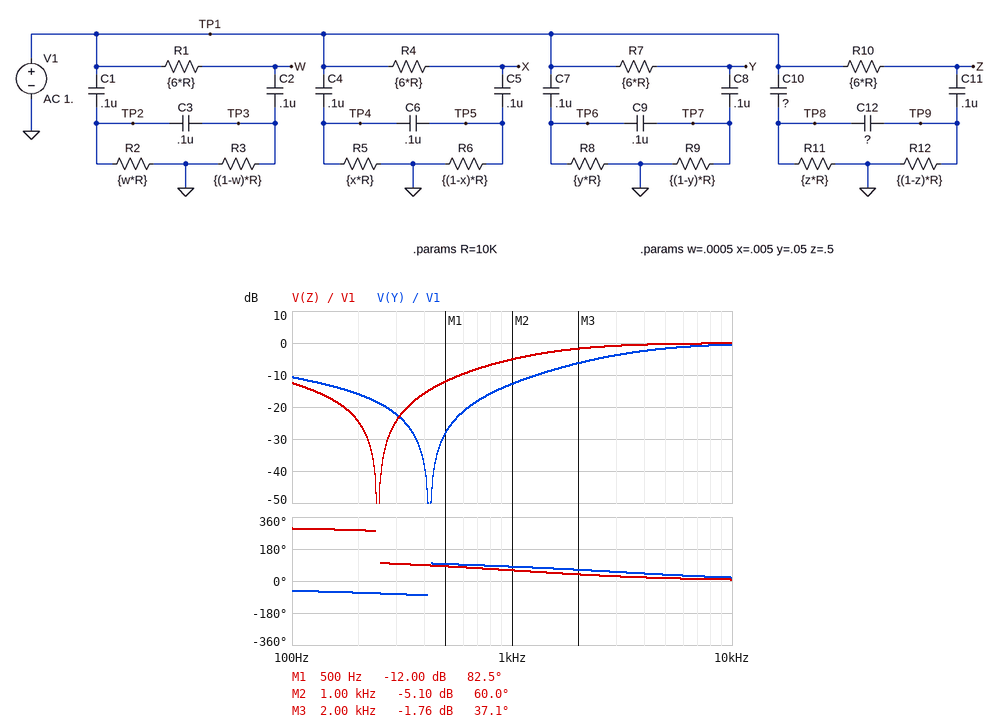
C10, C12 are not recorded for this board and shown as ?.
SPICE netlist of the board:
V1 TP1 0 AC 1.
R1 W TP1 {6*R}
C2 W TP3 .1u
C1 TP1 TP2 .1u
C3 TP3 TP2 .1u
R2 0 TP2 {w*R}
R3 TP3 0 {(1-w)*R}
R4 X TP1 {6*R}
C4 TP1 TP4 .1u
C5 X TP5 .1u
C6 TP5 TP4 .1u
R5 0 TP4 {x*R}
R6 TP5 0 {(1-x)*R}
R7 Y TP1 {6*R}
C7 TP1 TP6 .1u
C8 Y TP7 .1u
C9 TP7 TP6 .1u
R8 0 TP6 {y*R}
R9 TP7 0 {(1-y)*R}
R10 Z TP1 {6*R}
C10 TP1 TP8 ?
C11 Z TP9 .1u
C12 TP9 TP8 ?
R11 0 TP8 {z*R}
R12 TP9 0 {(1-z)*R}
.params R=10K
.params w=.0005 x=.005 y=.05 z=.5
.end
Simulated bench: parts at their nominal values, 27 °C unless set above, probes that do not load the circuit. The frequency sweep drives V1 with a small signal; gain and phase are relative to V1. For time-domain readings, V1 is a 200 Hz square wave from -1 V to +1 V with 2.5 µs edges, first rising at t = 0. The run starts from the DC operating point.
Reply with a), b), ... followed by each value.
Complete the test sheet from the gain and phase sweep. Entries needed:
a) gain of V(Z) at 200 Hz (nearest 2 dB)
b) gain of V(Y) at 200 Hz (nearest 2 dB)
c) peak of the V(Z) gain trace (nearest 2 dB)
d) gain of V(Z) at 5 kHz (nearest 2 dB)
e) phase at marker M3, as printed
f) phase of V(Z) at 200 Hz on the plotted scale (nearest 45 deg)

a) -24 dB
b) -16 dB
c) 0 dB
d) 0 dB
e) 37.1 deg
f) 270 deg
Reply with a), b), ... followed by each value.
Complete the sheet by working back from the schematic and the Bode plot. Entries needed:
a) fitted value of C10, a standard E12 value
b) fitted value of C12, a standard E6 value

a) 82 nF
b) 47 nF
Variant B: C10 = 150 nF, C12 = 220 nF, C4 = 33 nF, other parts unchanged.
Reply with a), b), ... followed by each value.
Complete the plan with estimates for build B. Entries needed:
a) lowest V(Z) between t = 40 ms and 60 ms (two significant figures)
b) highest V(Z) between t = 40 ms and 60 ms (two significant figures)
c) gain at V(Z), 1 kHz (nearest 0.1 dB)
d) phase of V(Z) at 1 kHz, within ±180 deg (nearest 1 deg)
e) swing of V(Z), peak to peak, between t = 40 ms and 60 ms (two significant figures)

a) -1.8 V
b) 1.8 V
c) -1.3 dB
d) 30 deg
e) 3.7 V
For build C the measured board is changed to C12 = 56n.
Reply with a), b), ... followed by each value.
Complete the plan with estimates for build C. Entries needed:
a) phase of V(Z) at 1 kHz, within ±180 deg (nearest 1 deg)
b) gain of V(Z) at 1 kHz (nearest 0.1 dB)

a) 57 deg
b) -4.6 dB
